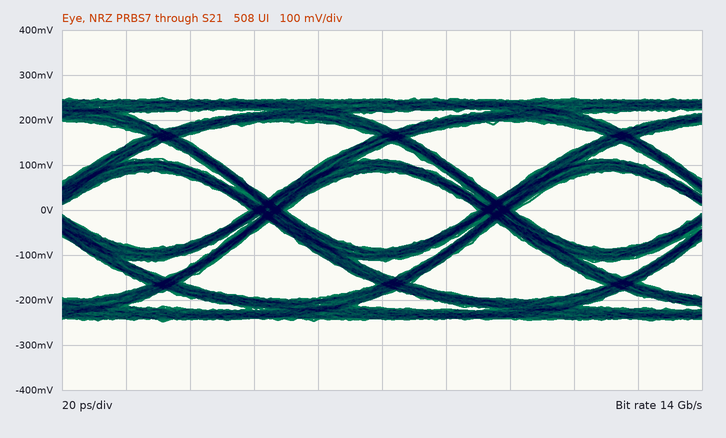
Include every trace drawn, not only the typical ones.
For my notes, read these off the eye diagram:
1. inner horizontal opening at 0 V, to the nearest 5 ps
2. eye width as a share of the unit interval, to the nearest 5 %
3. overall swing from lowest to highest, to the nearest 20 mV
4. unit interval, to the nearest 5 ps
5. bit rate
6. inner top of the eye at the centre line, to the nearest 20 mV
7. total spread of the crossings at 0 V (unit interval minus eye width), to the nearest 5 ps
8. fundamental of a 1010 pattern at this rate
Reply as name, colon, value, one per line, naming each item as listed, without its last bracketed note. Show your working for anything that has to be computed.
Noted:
inner horizontal opening at 0 V, to the nearest 5 ps: 60 ps
eye width as a share of the unit interval, to the nearest 5 %: 60 ps / 70 ps ≈ 85.7 %, so 85 % to the nearest 5 %
overall swing from lowest to highest, to the nearest 20 mV: 500 mV
unit interval, to the nearest 5 ps: 70 ps
bit rate: 14 Gb/s
inner top of the eye at the centre line, to the nearest 20 mV: 80 mV
total spread of the crossings at 0 V (unit interval minus eye width), to the nearest 5 ps: 10 ps
fundamental of a 1010 pattern at this rate: 7 GHz
